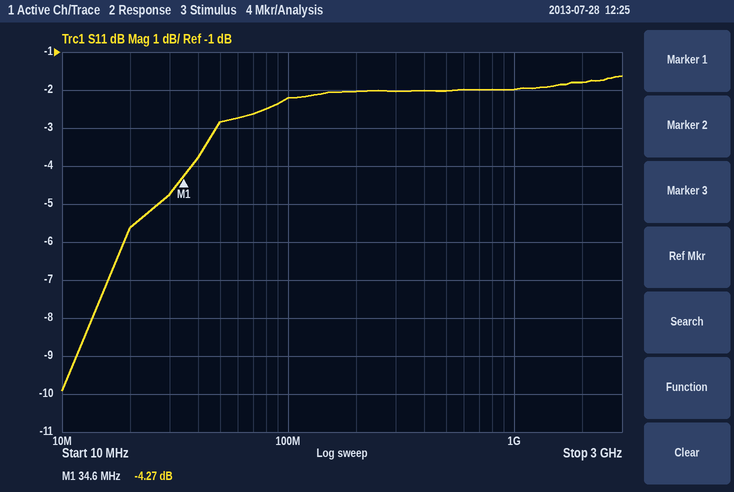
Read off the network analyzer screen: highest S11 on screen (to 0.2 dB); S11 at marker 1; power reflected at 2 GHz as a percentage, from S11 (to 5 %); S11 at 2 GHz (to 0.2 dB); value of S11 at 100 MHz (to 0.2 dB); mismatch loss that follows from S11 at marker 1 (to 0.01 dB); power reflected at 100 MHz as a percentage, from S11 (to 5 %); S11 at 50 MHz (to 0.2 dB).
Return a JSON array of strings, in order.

["-1.6 dB", "-4.27 dB", "65 %", "-1.8 dB", "-2.2 dB", "2.04 dB", "60 %", "-2.8 dB"]
